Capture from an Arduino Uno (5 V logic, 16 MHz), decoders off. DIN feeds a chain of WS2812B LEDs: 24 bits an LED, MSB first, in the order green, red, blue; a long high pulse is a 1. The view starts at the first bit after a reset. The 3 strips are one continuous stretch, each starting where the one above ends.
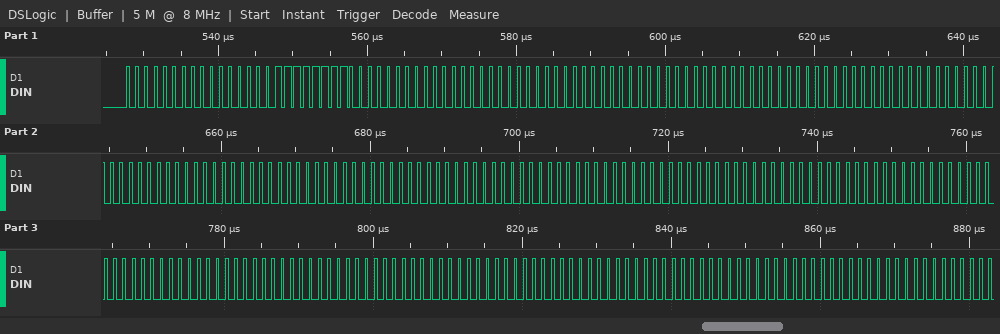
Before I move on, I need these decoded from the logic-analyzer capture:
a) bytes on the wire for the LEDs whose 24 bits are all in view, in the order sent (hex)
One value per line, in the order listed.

00 00 FF 00 00 00 00 00 00 00 00 00 00 00 00 00 00 00 00 00 00 00 00 00 00 00 00 00 00 00 00 00 00
